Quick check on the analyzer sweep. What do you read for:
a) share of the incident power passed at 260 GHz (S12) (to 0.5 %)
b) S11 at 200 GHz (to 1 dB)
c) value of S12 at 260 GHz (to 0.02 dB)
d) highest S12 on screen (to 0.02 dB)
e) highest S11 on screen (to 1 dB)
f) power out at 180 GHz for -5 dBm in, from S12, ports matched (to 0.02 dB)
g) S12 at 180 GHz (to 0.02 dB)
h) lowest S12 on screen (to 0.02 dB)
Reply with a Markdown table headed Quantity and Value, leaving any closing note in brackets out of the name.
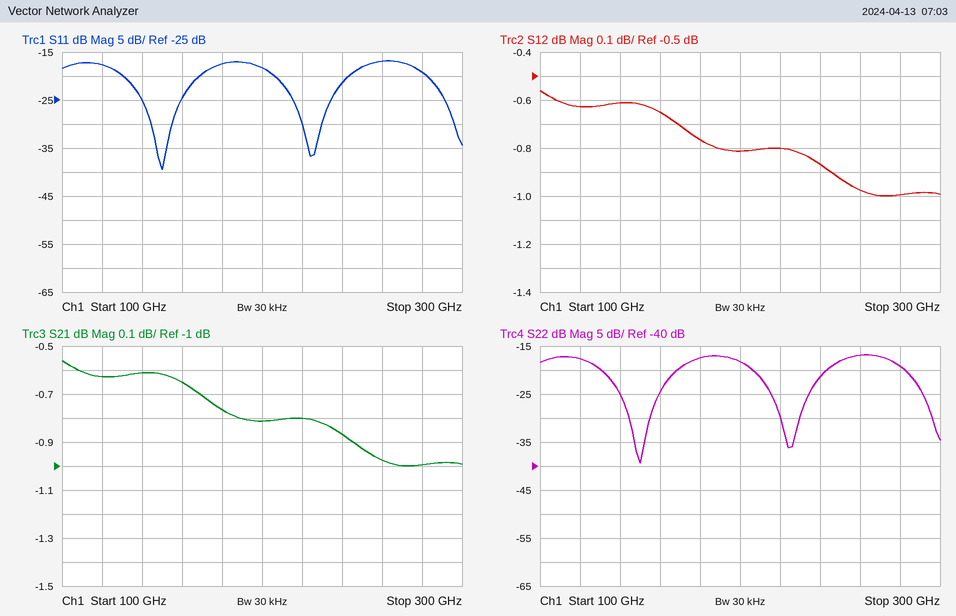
| Quantity | Value |
|---|---|
| share of the incident power passed at 260 GHz (S12) | 80.0 % |
| S11 at 200 GHz | -18 dB |
| value of S12 at 260 GHz | -0.98 dB |
| highest S12 on screen | -0.56 dB |
| highest S11 on screen | -17 dB |
| power out at 180 GHz for -5 dBm in, from S12, ports matched | -5.76 dBm |
| S12 at 180 GHz | -0.76 dB |
| lowest S12 on screen | -1.00 dB |
